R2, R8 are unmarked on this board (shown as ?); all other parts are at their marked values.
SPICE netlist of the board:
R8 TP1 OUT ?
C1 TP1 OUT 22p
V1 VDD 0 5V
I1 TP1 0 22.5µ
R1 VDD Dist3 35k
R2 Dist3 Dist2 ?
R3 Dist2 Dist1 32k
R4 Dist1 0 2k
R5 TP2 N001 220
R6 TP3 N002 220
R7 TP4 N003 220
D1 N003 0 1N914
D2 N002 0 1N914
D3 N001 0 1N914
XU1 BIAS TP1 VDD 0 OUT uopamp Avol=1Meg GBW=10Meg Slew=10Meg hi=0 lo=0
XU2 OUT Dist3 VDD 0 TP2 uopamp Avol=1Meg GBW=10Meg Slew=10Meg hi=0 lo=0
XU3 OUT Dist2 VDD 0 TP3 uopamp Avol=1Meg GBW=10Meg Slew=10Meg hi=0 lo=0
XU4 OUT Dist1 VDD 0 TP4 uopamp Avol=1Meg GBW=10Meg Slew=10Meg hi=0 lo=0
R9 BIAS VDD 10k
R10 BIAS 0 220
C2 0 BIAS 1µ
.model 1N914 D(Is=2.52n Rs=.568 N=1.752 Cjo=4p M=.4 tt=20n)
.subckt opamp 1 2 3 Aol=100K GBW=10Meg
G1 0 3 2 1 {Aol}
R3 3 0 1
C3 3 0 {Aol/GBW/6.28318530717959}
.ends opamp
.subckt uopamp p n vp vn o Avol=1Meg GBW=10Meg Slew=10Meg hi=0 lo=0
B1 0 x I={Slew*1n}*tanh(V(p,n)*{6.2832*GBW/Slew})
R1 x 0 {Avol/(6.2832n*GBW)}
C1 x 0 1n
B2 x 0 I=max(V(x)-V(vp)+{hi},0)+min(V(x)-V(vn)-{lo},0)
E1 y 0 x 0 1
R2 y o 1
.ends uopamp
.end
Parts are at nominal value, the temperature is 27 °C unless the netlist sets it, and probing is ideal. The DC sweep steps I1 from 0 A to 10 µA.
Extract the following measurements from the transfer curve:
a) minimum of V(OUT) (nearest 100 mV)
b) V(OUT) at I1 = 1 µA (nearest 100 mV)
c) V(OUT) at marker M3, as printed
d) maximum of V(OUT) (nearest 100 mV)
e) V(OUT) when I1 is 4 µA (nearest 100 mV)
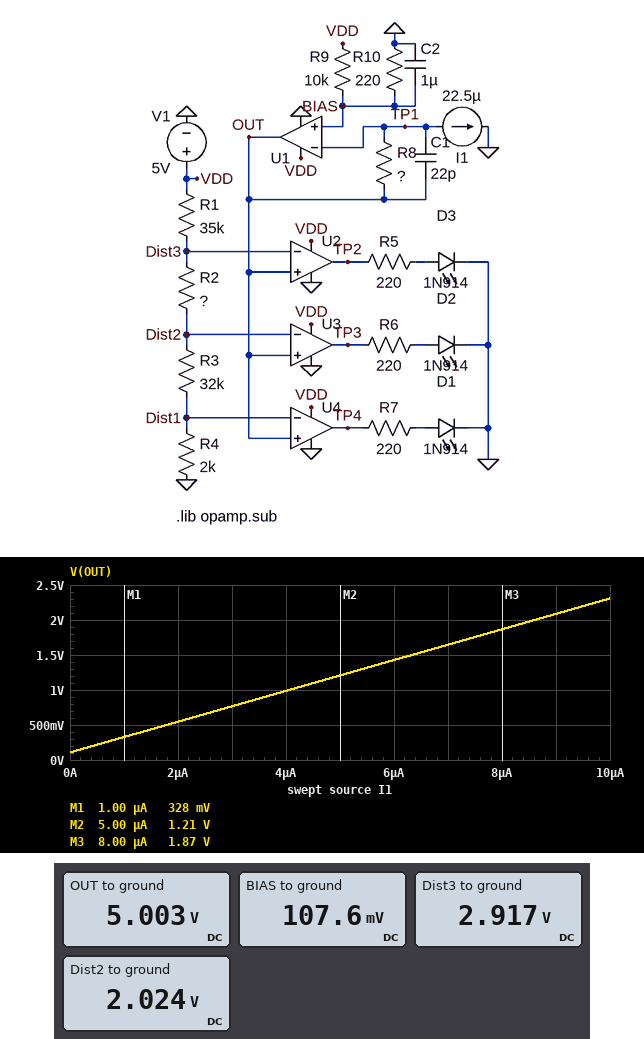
100 mV
300 mV
1.87 V
2.3 V
1.0 V
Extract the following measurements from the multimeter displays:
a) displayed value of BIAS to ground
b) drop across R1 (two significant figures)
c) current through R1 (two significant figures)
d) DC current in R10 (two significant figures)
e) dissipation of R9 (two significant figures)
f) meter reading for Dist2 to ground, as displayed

107.6 mV
2.1 V
60 µA
490 µA
2.4 mW
2.024 V
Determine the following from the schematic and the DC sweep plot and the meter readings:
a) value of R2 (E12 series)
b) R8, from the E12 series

15 kΩ
220 kΩ
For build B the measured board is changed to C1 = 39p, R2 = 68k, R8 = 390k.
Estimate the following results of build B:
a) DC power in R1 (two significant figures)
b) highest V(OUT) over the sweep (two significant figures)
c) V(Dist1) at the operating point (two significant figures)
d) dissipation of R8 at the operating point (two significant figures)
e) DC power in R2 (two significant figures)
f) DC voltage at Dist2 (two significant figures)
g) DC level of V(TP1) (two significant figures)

47 µW
4.0 V
73 mV
200 µW
91 µW
1.2 V
-3.8 V
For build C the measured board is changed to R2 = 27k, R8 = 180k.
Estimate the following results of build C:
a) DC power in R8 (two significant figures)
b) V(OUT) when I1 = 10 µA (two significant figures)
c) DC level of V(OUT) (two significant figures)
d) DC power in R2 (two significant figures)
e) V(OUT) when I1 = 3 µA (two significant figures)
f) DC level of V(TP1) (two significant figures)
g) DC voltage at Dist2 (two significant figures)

91 µW
1.9 V
4.2 V
73 µW
650 mV
110 mV
1.8 V
